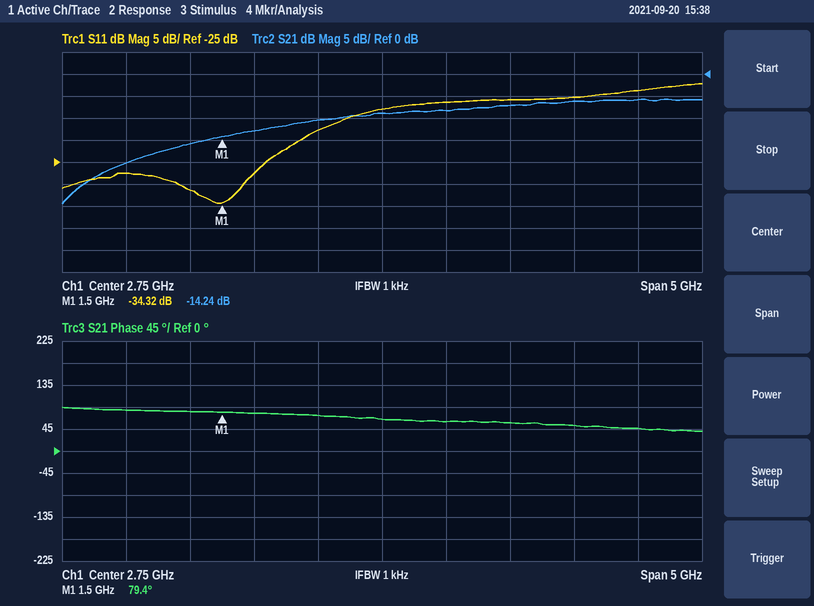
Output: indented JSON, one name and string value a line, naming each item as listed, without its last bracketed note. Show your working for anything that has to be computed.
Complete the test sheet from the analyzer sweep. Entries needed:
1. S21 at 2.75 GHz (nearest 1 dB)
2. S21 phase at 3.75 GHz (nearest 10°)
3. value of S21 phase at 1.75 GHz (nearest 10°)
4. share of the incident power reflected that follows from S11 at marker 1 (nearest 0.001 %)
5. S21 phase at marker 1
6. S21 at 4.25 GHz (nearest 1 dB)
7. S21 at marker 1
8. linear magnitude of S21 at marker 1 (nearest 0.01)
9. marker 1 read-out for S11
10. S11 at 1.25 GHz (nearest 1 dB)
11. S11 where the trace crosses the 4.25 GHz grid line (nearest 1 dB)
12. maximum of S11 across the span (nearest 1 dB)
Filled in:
{
  "S21 at 2.75 GHz": "-9 dB",
  "S21 phase at 3.75 GHz": "60°",
  "value of S21 phase at 1.75 GHz": "80°",
  "share of the incident power reflected that follows from S11 at marker 1": "10^(-34.32/10) ≈ 0.037 %",
  "S21 phase at marker 1": "79.4°",
  "S21 at 4.25 GHz": "-6 dB",
  "S21 at marker 1": "-14.24 dB",
  "linear magnitude of S21 at marker 1": "10^(-14.24/20) ≈ 0.19",
  "marker 1 read-out for S11": "-34.32 dB",
  "S11 at 1.25 GHz": "-31 dB",
  "S11 where the trace crosses the 4.25 GHz grid line": "-10 dB",
  "maximum of S11 across the span": "-7 dB"
}
